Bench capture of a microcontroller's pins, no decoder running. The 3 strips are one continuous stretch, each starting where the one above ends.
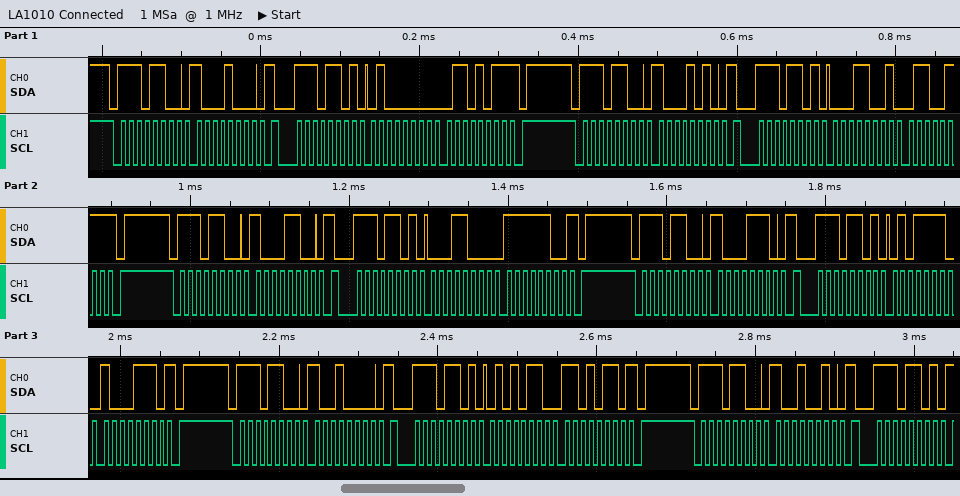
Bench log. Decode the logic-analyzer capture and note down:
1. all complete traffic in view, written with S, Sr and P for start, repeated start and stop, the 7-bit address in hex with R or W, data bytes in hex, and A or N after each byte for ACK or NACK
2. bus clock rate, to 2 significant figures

S 76W A 88 A Sr 76R A 40 A 6B N P S 76W A 8A A Sr 76R A 19 A 67 N P S 76W A 8C A Sr 76R A 18 A FC N P S 76W A 8E A Sr 76R A 5E A 8E N P S 76W A 90 A Sr 76R A 56 A D6 N P S 76W A 92 A Sr 76R A
100 kHz
